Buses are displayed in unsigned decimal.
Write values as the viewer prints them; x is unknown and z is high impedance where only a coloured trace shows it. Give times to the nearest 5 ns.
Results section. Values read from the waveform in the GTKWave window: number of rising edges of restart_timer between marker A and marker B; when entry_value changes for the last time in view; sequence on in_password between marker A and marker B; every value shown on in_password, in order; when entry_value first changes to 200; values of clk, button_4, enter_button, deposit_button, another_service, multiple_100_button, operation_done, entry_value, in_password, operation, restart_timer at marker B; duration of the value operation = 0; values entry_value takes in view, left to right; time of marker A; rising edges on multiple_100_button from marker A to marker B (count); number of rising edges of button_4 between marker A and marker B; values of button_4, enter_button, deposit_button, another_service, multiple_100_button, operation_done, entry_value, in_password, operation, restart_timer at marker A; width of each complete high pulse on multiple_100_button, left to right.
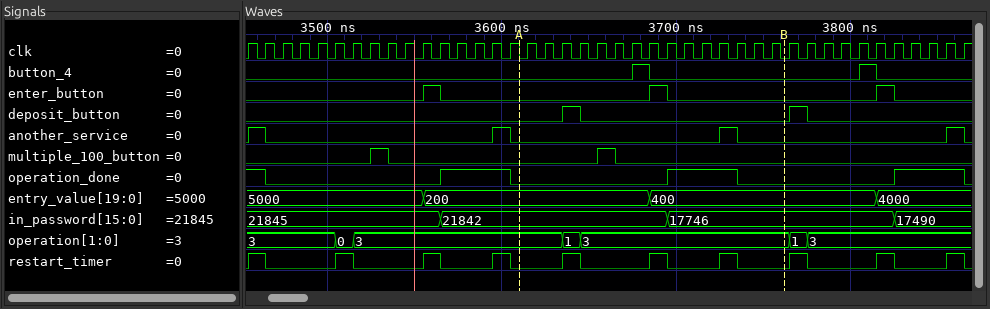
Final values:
3
3815 ns
21842, 17746
21845, 21842, 17746, 17490
3555 ns
clk=0, button_4=0, enter_button=0, deposit_button=0, another_service=0, multiple_100_button=0, operation_done=0, entry_value=400, in_password=17746, operation=3, restart_timer=0
10 ns
5000, 200, 400, 4000
3610 ns
1
1
button_4=0, enter_button=0, deposit_button=0, another_service=0, multiple_100_button=0, operation_done=0, entry_value=200, in_password=21842, operation=3, restart_timer=0
10 ns, 10 ns
